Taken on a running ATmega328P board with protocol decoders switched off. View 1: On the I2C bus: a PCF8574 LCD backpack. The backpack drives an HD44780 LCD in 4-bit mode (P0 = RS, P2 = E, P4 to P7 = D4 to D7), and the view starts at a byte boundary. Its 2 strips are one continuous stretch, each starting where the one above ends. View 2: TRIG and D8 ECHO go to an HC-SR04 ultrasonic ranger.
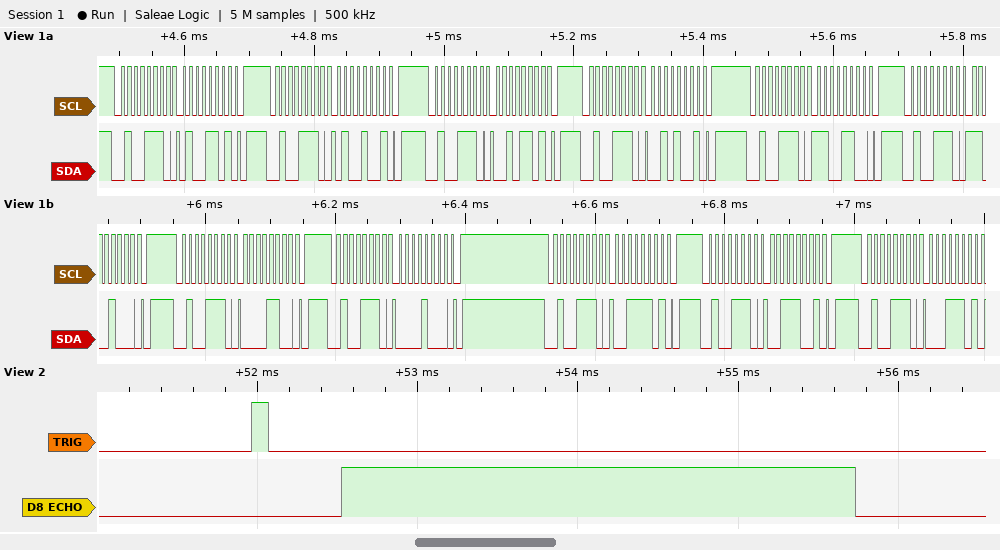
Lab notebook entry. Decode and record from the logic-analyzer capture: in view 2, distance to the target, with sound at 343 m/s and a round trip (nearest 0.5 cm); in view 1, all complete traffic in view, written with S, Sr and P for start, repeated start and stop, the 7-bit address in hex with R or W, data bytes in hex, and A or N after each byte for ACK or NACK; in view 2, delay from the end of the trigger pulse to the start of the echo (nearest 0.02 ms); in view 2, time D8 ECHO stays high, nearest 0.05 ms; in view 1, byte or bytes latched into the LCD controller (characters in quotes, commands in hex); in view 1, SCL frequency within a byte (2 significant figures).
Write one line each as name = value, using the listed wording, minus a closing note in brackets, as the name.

in view 2, distance to the target, with sound at 343 m/s and a round trip = 55 cm
in view 1, all complete traffic in view, written with S, Sr and P for start, repeated start and stop, the 7-bit address in hex with R or W, data bytes in hex, and A or N after each byte for ACK or NACK = S 27W A 4D A P S 27W A 49 A P S 27W A 2D A P S 27W A 29 A P S 27W A CC A P S 27W A C8 A P S 27W A 0C A P S 27W A 08 A P S 27W A 3D A P S 27W A 39 A P S 27W A 1D A
in view 2, delay from the end of the trigger pulse to the start of the echo = 0.46 ms
in view 2, time D8 ECHO stays high, nearest 0.05 ms = 3.20 ms
in view 1, byte or bytes latched into the LCD controller = 'B' 0xC0
in view 1, SCL frequency within a byte = 100 kHz
